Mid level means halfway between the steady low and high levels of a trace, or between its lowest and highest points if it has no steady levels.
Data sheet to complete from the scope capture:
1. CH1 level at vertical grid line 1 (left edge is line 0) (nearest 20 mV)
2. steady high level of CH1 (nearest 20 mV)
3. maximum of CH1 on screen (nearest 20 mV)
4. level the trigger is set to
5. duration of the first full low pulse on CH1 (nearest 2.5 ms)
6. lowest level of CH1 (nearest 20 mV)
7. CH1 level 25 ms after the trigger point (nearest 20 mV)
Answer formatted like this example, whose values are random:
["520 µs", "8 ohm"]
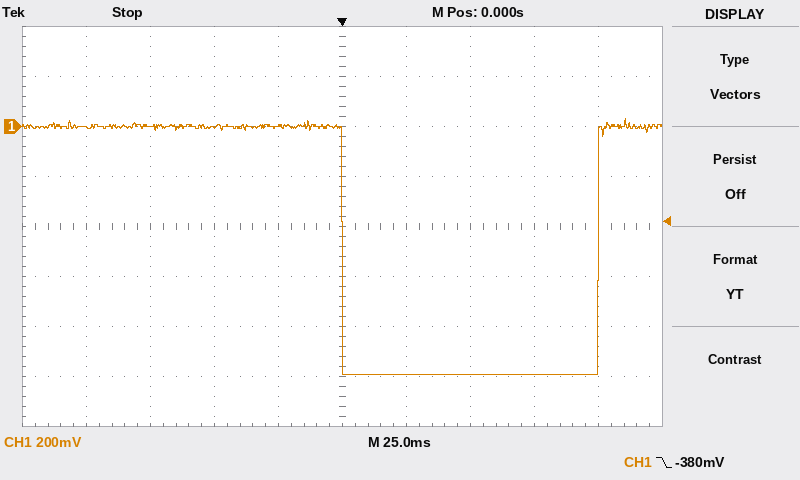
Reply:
["0 mV", "0 mV", "40 mV", "-380 mV", "100.0 ms", "-1.00 V", "-1.00 V"]
